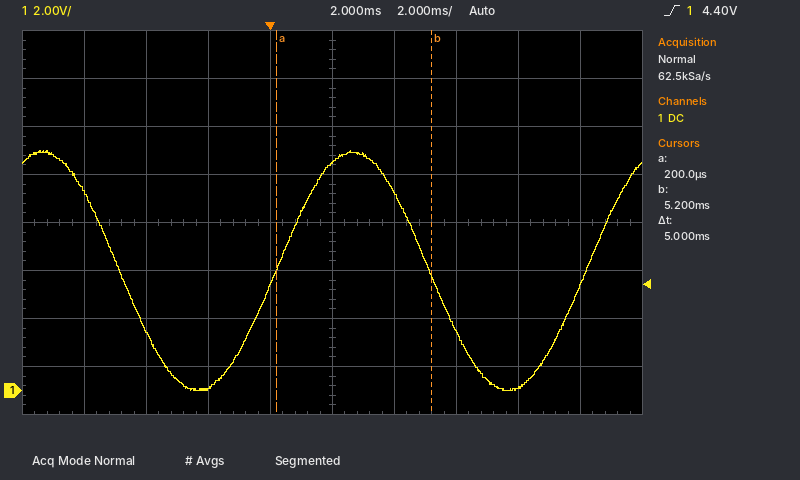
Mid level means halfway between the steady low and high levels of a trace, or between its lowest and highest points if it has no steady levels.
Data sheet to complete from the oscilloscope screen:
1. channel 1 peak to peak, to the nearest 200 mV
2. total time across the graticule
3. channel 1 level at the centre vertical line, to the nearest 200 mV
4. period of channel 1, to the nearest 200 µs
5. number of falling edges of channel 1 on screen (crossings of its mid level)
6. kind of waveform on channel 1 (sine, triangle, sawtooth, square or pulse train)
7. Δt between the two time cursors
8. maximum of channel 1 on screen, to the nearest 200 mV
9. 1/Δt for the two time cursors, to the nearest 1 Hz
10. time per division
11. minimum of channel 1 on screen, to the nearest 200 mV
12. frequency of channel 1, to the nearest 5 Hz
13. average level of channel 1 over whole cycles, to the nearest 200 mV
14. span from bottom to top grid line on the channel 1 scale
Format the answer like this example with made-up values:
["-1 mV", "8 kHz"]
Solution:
["10.0 V", "20 ms", "9.4 V", "10.0 ms", "2", "sine", "5 ms", "10.0 V", "200 Hz", "2 ms", "0.0 V", "100 Hz", "5.0 V", "16 V"]
